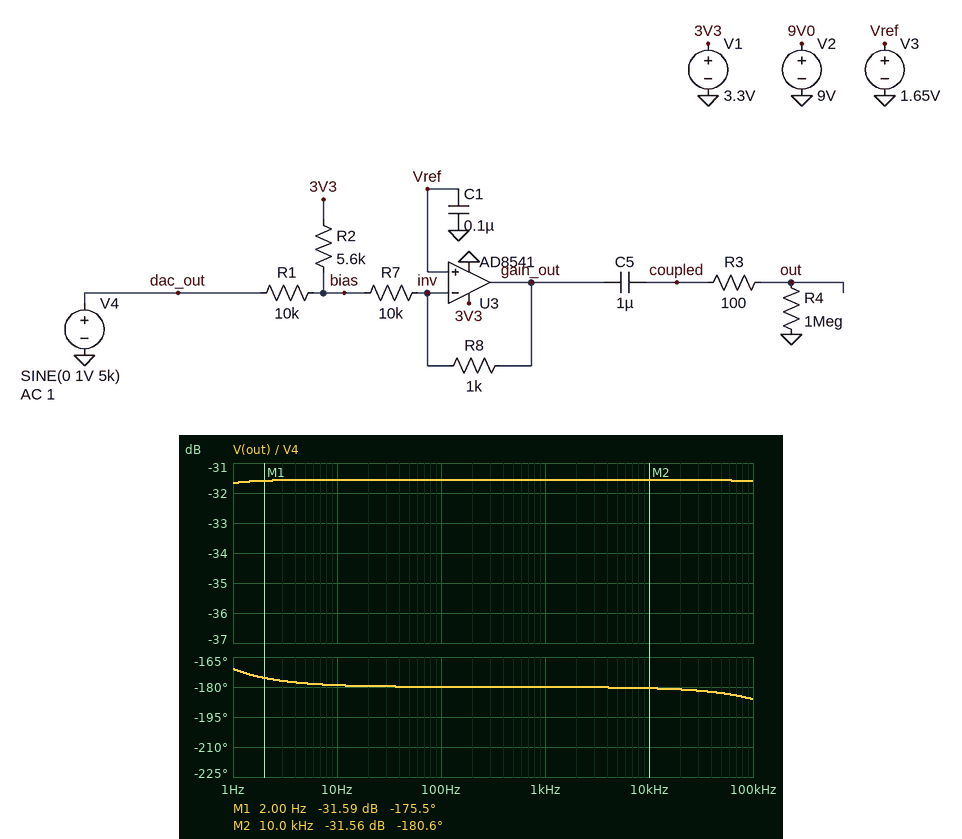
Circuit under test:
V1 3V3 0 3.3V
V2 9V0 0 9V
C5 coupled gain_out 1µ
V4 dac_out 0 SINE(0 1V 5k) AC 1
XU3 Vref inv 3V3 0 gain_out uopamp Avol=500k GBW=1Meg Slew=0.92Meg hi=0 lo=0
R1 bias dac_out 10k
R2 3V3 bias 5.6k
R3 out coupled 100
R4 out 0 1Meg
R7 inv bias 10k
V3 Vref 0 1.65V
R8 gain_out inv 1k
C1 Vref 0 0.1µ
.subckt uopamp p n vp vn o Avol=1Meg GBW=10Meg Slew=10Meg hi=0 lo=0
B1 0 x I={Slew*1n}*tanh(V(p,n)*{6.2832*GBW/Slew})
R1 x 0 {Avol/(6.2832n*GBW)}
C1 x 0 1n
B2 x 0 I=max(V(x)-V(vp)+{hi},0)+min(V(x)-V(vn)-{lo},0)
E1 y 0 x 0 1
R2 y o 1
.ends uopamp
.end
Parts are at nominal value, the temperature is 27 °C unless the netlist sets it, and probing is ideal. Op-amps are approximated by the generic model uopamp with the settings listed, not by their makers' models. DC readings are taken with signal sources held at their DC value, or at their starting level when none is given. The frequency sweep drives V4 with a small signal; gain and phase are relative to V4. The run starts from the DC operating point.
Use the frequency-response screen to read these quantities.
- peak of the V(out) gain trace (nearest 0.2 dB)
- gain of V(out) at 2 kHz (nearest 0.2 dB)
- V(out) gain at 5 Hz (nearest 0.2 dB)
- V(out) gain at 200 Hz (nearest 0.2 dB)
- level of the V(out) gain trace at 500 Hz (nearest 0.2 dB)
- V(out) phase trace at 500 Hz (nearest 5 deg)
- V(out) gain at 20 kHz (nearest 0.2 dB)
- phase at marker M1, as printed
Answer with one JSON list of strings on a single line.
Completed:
["-31.6 dB", "-31.6 dB", "-31.6 dB", "-31.6 dB", "-31.6 dB", "-180 deg", "-31.6 dB", "-175.5 deg"]
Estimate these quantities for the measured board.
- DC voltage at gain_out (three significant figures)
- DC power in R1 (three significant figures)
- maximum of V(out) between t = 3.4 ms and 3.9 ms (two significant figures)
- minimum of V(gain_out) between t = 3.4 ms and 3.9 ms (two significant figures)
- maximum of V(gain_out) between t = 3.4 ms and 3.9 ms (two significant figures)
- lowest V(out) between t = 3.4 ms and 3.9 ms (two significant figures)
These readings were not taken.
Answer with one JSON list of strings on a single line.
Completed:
["1.62 V", "397 µW", "26 mV", "1.6 V", "1.6 V", "-26 mV"]
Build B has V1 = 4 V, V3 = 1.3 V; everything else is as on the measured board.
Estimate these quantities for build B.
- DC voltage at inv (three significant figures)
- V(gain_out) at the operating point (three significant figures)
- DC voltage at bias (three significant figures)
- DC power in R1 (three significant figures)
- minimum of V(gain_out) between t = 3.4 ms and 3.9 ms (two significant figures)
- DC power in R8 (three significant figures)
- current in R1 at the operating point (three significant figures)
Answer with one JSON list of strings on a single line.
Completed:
["1.30 V", "1.21 V", "2.23 V", "497 µW", "1.2 V", "8.65 µW", "223 µA"]
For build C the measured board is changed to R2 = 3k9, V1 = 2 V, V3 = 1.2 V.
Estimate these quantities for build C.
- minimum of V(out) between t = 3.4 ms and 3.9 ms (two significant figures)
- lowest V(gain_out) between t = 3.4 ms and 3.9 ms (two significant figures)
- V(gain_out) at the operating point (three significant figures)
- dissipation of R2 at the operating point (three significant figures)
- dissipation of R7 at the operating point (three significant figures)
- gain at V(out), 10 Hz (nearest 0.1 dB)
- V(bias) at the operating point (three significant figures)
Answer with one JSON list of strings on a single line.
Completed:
["-22 mV", "1.2 V", "1.18 V", "96.5 µW", "3.48 µW", "-33.2 dB", "1.39 V"]
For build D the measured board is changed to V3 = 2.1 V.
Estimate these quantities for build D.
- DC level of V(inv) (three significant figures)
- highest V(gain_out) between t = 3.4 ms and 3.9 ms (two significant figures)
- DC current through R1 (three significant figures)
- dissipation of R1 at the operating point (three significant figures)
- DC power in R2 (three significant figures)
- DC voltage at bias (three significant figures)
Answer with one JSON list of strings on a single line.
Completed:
["2.10 V", "2.1 V", "211 µA", "446 µW", "252 µW", "2.11 V"]
